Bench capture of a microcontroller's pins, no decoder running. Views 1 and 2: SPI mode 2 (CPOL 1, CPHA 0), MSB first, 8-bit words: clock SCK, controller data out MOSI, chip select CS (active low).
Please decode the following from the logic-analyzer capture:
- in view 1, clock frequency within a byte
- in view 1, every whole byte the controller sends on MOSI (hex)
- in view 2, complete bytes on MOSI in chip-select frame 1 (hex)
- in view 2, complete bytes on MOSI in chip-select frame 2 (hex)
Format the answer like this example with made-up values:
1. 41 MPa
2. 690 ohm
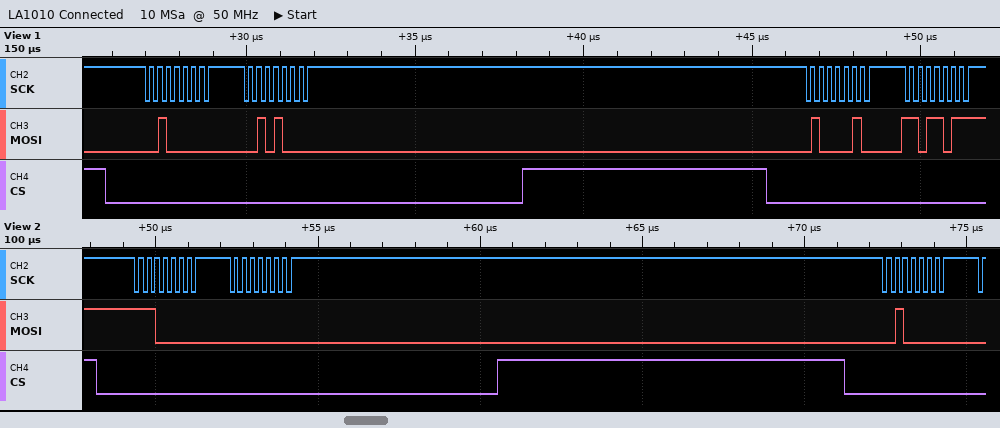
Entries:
1. 4 MHz
2. 20 28 42 DB
3. E0 00
4. 20
